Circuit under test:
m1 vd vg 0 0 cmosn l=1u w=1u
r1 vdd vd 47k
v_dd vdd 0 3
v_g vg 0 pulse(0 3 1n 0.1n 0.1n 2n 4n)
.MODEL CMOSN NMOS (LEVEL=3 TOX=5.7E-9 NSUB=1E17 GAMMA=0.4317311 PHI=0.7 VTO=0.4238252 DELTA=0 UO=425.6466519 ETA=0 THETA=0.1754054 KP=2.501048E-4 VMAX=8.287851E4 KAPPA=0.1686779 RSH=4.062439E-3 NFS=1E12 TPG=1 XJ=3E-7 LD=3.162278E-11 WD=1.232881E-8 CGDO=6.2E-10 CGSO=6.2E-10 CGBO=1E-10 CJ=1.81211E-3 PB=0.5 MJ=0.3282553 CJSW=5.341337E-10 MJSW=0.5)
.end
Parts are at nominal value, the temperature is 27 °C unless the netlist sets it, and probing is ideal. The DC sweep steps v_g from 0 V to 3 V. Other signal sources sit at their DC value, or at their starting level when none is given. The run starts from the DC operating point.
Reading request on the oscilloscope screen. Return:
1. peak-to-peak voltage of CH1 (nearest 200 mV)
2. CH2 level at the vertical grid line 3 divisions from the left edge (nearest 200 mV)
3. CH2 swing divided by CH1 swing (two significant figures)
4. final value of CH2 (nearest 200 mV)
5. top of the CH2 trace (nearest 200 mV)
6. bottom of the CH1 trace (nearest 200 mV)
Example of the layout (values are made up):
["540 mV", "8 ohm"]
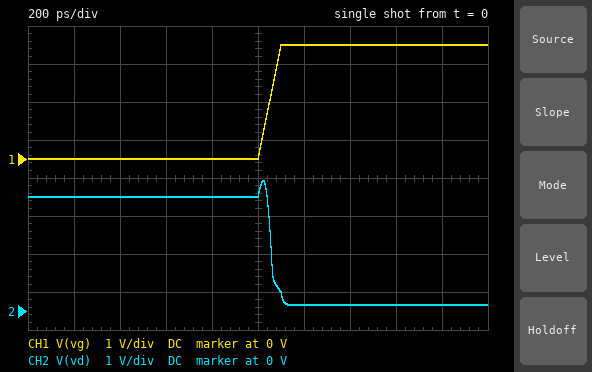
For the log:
["3.0 V", "3.0 V", "1.1", "200 mV", "3.4 V", "0 V"]
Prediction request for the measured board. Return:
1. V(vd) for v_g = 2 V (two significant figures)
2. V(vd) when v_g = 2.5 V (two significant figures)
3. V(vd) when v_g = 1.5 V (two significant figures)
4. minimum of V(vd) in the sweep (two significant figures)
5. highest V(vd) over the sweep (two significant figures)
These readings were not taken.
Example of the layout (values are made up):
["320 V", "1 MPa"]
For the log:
["230 mV", "180 mV", "350 mV", "150 mV", "3.0 V"]
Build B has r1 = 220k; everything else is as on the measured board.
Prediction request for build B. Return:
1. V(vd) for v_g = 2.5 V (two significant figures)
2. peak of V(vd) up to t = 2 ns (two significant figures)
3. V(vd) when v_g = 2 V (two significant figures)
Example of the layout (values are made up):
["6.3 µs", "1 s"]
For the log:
["37 mV", "3.6 V", "45 mV"]
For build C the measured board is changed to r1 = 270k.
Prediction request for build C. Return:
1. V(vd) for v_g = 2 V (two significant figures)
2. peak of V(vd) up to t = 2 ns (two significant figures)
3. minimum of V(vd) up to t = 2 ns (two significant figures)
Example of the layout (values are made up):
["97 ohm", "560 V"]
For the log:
["37 mV", "3.6 V", "26 mV"]
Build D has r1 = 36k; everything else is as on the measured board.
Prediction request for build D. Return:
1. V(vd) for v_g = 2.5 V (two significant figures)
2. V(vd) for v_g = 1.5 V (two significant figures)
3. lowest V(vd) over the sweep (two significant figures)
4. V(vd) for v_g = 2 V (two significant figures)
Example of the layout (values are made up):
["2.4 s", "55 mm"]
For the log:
["240 mV", "500 mV", "200 mV", "310 mV"]
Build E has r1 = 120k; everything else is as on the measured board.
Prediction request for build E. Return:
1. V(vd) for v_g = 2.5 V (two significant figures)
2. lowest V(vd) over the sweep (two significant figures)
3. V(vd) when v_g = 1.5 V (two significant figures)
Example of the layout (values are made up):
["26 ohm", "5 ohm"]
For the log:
["68 mV", "58 mV", "120 mV"]
